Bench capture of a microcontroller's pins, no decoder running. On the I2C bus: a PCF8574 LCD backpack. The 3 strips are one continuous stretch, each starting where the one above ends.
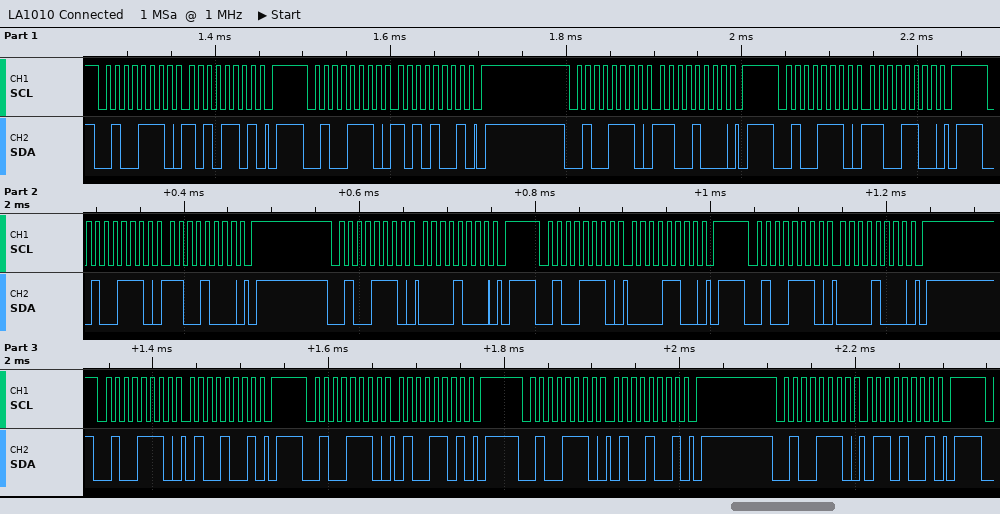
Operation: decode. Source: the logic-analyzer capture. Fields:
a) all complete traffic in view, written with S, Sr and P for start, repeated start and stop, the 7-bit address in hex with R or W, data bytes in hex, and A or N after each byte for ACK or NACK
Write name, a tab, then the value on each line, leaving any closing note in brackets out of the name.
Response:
all complete traffic in view, written with S, Sr and P for start, repeated start and stop, the 7-bit address in hex with R or W, data bytes in hex, and A or N after each byte for ACK or NACK	S 27W A AD A P S 27W A A9 A P S 27W A C8 A P S 27W A CC A P S 27W A C8 A P S 27W A 08 A P S 27W A 0C A P S 27W A 08 A P S 27W A 49 A P S 27W A 4D A P S 27W A 49 A P S 27W A 69 A P
